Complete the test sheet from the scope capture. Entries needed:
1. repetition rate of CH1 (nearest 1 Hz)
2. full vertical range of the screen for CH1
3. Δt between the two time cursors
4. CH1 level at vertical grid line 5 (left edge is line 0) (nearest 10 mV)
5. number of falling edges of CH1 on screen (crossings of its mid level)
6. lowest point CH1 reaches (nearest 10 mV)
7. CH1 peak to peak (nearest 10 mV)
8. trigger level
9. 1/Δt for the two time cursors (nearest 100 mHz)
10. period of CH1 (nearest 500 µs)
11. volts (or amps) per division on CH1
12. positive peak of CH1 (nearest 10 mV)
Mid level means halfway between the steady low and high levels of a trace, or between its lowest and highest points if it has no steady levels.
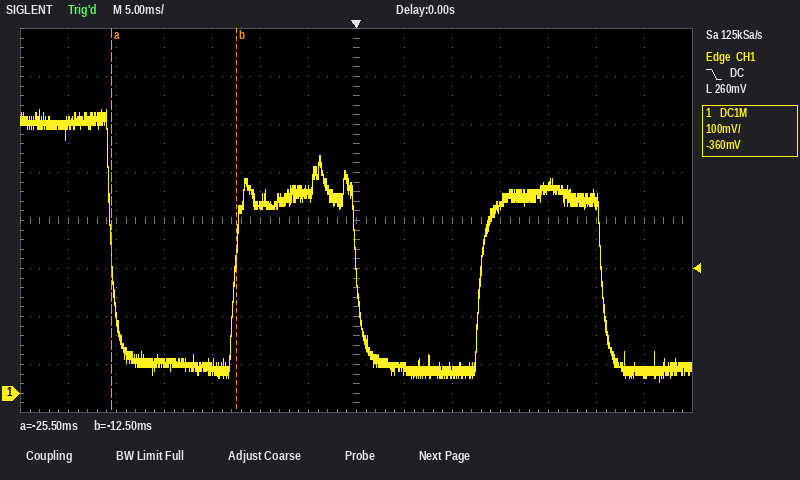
39 Hz
800 mV
13.0 ms
390 mV
3
20 mV
570 mV
260 mV
76.9 Hz
25.5 ms
100 mV
590 mV
